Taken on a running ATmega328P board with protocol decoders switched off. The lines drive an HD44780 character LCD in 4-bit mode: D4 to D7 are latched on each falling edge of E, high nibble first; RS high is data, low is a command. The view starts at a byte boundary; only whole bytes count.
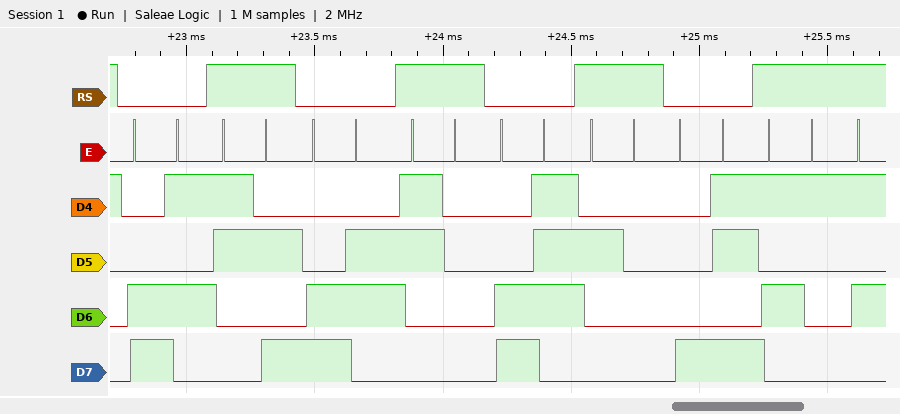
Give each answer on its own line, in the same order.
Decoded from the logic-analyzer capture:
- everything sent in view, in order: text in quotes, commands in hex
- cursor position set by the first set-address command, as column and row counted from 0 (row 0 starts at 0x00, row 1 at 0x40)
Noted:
0xC5 ":" 0xC6 "0" 0xC7 " " 0x8B "Q"
column 5, row 1
